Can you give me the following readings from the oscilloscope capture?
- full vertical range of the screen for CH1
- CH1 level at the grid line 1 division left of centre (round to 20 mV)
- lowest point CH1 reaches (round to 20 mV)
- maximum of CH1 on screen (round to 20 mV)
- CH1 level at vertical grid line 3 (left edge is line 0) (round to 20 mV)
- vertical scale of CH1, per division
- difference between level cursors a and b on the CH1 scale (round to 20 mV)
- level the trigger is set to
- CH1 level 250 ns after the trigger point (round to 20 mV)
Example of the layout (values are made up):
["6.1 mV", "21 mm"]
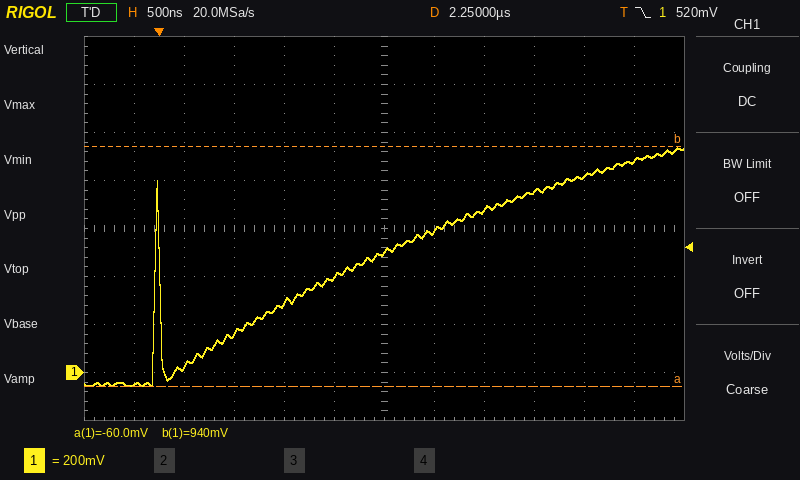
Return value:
["1.6 V", "400 mV", "-60 mV", "940 mV", "160 mV", "200 mV", "1.00 V", "520 mV", "20 mV"]
